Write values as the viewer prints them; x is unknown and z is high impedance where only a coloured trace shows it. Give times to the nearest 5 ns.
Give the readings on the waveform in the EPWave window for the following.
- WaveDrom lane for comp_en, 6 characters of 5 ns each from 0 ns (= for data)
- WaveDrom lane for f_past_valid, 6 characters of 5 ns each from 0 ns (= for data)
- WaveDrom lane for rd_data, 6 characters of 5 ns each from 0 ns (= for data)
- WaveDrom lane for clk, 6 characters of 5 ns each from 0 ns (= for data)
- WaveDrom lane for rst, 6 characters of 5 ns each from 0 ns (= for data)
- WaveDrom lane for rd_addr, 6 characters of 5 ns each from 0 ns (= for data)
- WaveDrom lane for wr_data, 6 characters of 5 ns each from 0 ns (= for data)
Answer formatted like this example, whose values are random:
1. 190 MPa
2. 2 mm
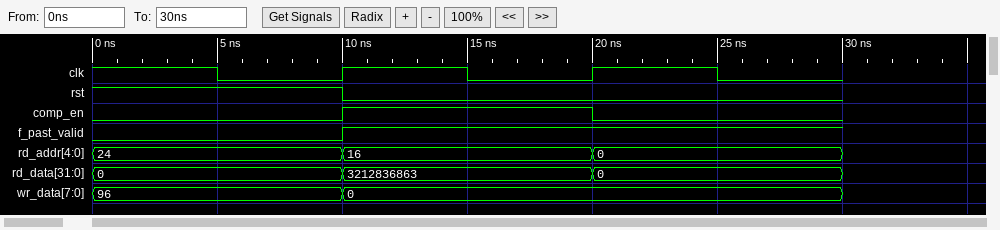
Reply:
1. {name: 'comp_en', wave: '0.1.0.'}
2. {name: 'f_past_valid', wave: '0.1...'}
3. {name: 'rd_data', wave: '=.=.=.', data: '0 3212836863 0'}
4. {name: 'clk', wave: '101010'}
5. {name: 'rst', wave: '1.0...'}
6. {name: 'rd_addr', wave: '=.=.=.', data: '24 16 0'}
7. {name: 'wr_data', wave: '=.=...', data: '96 0'}
